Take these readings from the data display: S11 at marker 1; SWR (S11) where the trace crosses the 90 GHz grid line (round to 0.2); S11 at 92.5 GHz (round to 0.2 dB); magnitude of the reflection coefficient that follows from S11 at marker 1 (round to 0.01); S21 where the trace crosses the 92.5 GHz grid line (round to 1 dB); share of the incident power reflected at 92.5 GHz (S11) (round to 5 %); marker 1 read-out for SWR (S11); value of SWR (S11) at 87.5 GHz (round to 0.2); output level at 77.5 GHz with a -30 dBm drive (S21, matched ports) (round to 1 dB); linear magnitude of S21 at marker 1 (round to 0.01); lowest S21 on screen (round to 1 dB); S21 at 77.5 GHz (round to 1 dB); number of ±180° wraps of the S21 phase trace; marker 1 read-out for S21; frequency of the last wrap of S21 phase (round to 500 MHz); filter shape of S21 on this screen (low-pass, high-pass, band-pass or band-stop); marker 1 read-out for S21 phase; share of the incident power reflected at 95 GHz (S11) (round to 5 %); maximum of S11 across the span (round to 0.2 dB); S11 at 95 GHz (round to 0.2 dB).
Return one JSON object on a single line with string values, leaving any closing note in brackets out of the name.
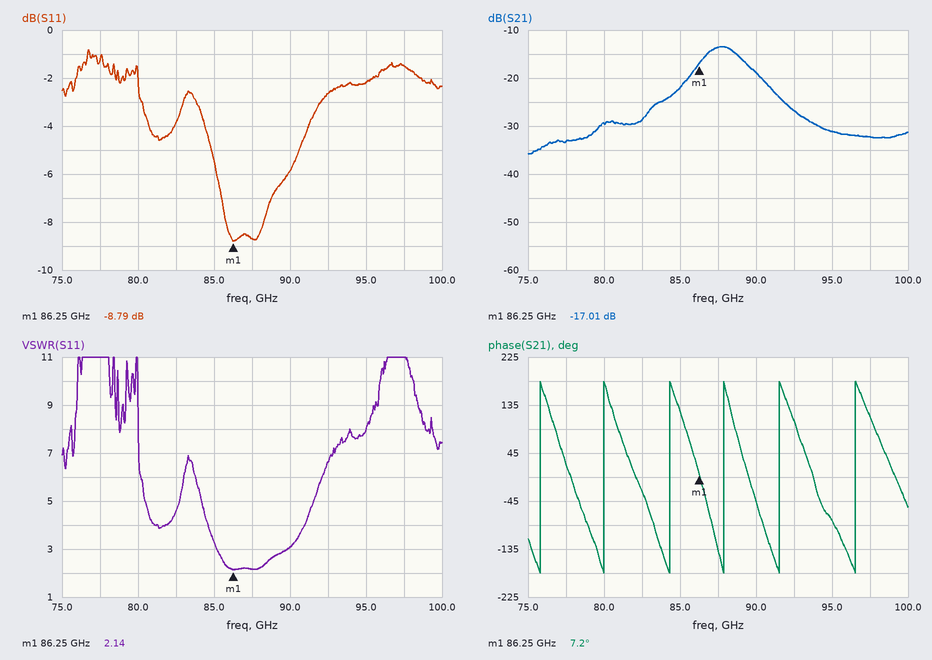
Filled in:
{"S11 at marker 1": "-8.79 dB", "SWR (S11) where the trace crosses the 90 GHz grid line": "3.0", "S11 at 92.5 GHz": "-2.6 dB", "magnitude of the reflection coefficient that follows from S11 at marker 1": "0.36", "S21 where the trace crosses the 92.5 GHz grid line": "-27 dB", "share of the incident power reflected at 92.5 GHz (S11)": "55 %", "marker 1 read-out for SWR": "2.14", "value of SWR (S11) at 87.5 GHz": "2.2", "output level at 77.5 GHz with a -30 dBm drive (S21, matched ports)": "-63 dBm", "linear magnitude of S21 at marker 1": "0.14", "lowest S21 on screen": "-36 dB", "S21 at 77.5 GHz": "-33 dB", "number of ±180° wraps of the S21 phase trace": "6", "marker 1 read-out for S21": "-17.01 dB", "frequency of the last wrap of S21 phase": "96.5 GHz", "filter shape of S21 on this screen": "band-pass", "marker 1 read-out for S21 phase": "7.2°", "share of the incident power reflected at 95 GHz (S11)": "60 %", "maximum of S11 across the span": "-0.8 dB", "S11 at 95 GHz": "-2.2 dB"}
